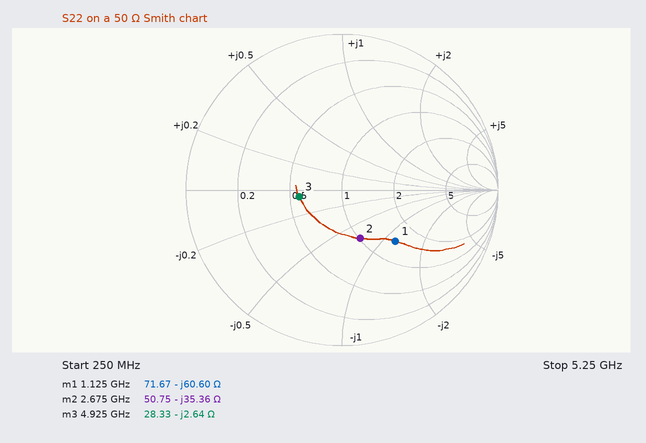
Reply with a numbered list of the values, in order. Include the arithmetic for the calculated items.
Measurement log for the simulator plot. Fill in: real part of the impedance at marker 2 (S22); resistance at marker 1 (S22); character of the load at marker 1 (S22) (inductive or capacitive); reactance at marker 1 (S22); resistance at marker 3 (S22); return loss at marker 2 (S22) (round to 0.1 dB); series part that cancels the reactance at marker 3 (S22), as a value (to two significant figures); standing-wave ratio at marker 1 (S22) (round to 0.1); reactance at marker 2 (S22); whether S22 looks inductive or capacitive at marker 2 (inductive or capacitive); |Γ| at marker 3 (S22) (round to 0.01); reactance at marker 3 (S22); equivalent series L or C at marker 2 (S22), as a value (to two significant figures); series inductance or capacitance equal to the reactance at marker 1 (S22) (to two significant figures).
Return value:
1. 50.75 Ω
2. 71.67 Ω
3. capacitive
4. -60.60 Ω
5. 28.33 Ω
6. 9.6 dB
7. L = 2.64 Ω/(2π × 4.925 GHz) ≈ 85 pH
8. 2.8
9. -35.36 Ω
10. capacitive
11. 0.28
12. -2.64 Ω
13. C = 1/(2π × 2.675 GHz × 35.36 Ω) ≈ 1.7 pF
14. C = 1/(2π × 1.125 GHz × 60.6 Ω) ≈ 2.3 pF
